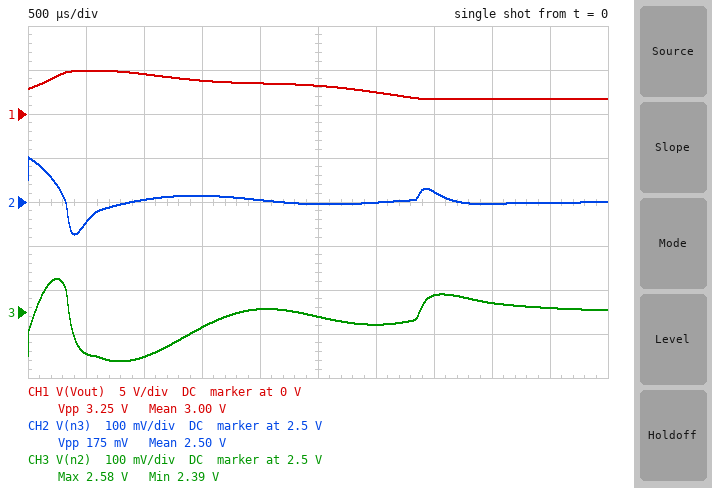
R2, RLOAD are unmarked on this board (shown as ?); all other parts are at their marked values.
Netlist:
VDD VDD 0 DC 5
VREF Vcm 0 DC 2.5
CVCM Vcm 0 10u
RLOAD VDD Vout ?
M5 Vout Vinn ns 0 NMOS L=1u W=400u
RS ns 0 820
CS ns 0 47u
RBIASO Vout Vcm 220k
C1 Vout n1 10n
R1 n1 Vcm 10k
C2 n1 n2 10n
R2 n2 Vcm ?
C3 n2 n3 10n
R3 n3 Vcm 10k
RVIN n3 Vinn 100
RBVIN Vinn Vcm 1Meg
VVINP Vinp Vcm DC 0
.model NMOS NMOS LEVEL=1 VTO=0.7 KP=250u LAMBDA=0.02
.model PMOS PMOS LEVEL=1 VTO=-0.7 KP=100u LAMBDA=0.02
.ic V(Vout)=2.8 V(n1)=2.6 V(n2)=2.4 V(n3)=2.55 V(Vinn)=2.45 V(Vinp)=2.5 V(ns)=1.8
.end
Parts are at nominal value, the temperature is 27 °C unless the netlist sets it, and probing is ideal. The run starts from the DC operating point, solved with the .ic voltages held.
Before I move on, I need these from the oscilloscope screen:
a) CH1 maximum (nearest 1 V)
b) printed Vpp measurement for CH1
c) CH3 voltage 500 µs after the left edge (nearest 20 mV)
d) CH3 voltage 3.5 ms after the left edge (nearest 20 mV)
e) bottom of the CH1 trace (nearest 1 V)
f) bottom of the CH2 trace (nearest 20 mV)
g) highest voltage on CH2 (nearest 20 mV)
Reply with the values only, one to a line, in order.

5 V
3.25 V
2.40 V
2.54 V
2 V
2.42 V
2.60 V
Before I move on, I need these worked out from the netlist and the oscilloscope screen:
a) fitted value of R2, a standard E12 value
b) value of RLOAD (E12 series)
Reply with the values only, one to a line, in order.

22 kΩ
3.9 kΩ
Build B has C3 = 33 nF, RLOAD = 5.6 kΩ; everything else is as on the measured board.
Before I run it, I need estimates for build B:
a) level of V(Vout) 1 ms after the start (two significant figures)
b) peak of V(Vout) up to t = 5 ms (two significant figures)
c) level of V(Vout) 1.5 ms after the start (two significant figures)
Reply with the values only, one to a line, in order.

4.7 V
4.8 V
3.7 V
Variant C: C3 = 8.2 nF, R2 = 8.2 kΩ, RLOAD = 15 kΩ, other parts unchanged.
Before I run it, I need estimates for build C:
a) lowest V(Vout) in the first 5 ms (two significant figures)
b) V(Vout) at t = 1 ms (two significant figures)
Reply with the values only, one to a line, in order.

1.6 V
4.1 V
